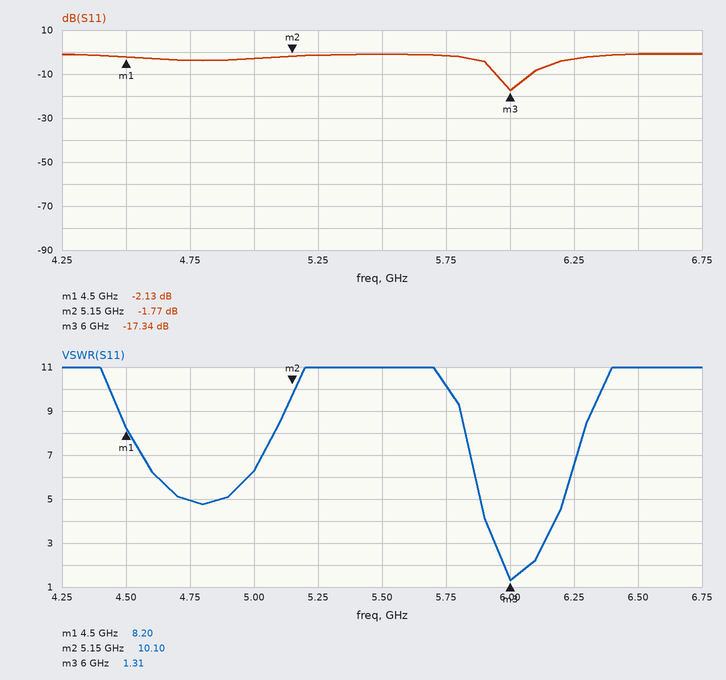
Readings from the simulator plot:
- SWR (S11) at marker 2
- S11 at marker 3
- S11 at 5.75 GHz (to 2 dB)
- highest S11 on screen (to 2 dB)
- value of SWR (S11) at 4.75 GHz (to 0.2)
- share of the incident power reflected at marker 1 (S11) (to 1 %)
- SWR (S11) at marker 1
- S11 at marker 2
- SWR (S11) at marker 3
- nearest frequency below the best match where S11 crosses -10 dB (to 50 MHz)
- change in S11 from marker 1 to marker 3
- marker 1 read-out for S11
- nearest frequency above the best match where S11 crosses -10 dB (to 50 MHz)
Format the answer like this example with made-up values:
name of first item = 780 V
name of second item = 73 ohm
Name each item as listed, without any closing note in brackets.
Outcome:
SWR (S11) at marker 2 = 10.10
S11 at marker 3 = -17.34 dB
S11 at 5.75 GHz = -2 dB
highest S11 on screen = 0 dB
value of SWR (S11) at 4.75 GHz = 5.0
share of the incident power reflected at marker 1 (S11) = 61 %
SWR (S11) at marker 1 = 8.20
S11 at marker 2 = -1.77 dB
SWR (S11) at marker 3 = 1.31
nearest frequency below the best match where S11 crosses -10 dB = 5.95 GHz
change in S11 from marker 1 to marker 3 = -15.21 dB
marker 1 read-out for S11 = -2.13 dB
nearest frequency above the best match where S11 crosses -10 dB = 6.10 GHz
